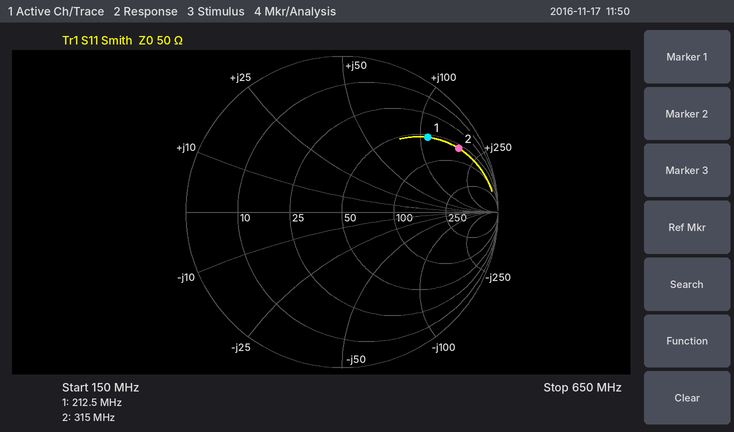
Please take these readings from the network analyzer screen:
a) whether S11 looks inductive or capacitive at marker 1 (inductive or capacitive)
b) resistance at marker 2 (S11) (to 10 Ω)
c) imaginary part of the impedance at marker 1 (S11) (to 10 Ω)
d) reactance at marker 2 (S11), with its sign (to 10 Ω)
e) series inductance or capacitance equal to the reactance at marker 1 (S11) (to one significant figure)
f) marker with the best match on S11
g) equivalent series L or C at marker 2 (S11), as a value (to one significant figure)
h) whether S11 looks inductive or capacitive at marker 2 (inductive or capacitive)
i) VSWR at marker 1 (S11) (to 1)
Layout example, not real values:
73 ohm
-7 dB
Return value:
inductive
60 Ω
+110 Ω
+180 Ω
80 nH
marker 1
90 nH
inductive
6
